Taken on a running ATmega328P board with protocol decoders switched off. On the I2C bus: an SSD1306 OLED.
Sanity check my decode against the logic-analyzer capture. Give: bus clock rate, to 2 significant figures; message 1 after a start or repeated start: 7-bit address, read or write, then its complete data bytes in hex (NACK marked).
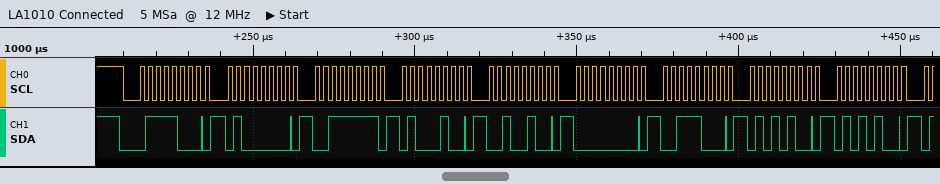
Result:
400 kHz
0x3C write: 40 3F 44 24 00 38 54 54
